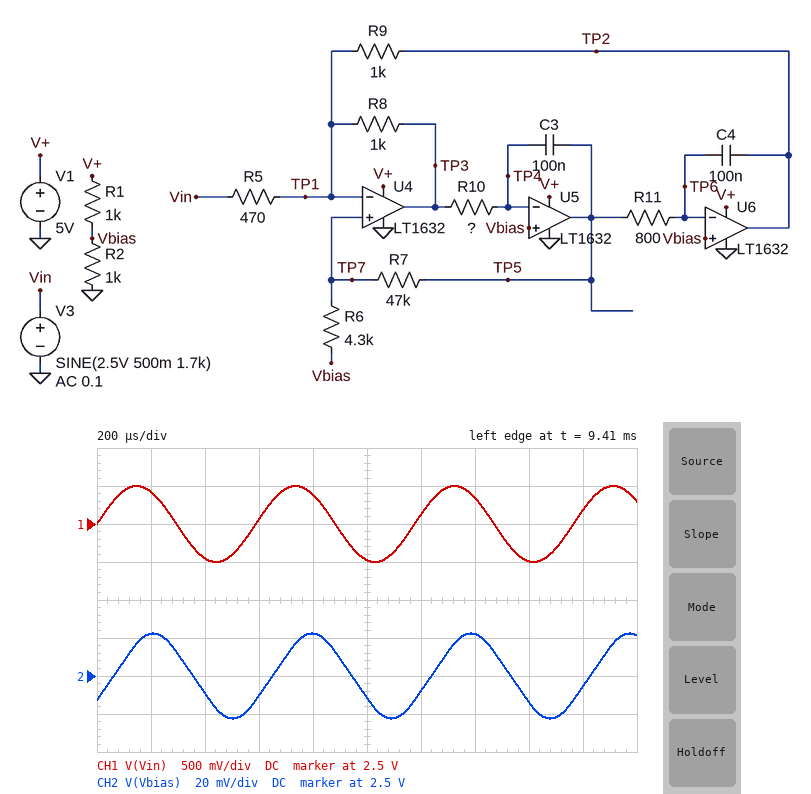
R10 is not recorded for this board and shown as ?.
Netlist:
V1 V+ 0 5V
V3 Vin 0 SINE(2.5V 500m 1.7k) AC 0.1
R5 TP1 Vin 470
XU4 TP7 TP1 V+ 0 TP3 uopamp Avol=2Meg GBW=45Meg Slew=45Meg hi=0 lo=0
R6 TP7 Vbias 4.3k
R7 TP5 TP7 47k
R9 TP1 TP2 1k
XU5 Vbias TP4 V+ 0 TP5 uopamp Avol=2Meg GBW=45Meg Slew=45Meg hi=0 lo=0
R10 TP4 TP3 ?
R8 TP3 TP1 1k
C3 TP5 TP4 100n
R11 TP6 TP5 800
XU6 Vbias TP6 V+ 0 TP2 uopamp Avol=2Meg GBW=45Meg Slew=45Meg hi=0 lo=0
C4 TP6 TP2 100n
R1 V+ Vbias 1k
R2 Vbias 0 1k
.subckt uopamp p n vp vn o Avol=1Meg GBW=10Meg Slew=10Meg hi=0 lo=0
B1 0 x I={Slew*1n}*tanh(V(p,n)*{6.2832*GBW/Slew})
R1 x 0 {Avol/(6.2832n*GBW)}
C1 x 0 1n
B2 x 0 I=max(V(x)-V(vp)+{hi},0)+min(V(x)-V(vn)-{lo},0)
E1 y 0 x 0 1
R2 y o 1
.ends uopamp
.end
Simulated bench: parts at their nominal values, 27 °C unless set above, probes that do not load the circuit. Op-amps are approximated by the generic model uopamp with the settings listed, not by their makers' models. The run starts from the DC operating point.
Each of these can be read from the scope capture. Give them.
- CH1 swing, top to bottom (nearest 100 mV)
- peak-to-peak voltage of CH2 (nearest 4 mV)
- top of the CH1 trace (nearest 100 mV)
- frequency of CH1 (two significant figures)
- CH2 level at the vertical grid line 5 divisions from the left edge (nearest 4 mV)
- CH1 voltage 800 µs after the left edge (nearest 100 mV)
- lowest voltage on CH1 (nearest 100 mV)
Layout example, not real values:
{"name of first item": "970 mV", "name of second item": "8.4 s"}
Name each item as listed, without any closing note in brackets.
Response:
{"CH1 swing, top to bottom": "1.0 V", "peak-to-peak voltage of CH2": "44 mV", "top of the CH1 trace": "3.0 V", "frequency of CH1": "1.7 kHz", "CH2 level at the vertical grid line 5 divisions from the left edge": "2.488 V", "CH1 voltage 800 µs after the left edge": "2.9 V", "lowest voltage on CH1": "2.0 V"}
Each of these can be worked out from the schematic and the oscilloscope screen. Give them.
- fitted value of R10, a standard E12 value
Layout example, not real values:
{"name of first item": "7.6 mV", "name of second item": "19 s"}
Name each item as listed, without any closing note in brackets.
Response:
{"fitted value of R10, a standard E12 value": "1.2 kΩ"}
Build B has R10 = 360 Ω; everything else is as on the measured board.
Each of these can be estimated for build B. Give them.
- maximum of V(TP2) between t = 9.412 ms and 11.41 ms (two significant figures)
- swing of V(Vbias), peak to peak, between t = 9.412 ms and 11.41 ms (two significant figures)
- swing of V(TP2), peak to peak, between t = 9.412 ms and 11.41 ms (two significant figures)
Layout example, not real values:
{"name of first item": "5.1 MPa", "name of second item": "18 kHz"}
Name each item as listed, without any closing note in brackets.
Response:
{"maximum of V(TP2) between t = 9.412 ms and 11.41 ms": "3.9 V", "swing of V(Vbias), peak to peak, between t = 9.412 ms and 11.41 ms": "24 mV", "swing of V(TP2), peak to peak, between t = 9.412 ms and 11.41 ms": "2.9 V"}
